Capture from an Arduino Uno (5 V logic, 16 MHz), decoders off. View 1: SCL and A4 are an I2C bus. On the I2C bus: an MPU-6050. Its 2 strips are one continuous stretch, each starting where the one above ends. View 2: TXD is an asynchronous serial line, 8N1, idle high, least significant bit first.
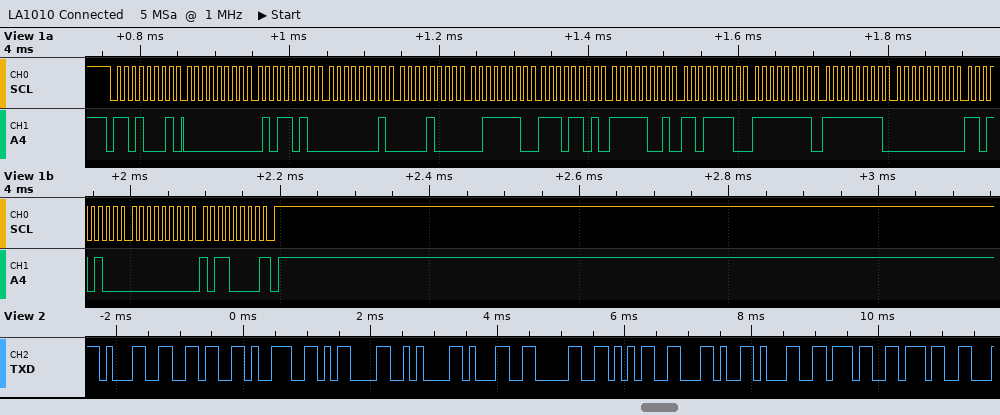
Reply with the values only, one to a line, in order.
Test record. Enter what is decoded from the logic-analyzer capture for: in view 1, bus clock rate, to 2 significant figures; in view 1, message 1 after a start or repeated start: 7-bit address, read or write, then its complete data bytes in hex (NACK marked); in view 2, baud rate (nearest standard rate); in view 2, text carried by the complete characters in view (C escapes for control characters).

100 kHz
0x68 read: 00 5A 01 08 3E ED F9 DE FF FF 00 D4 00 B0 NACK
9600 baud
"169\r\n105,177"
